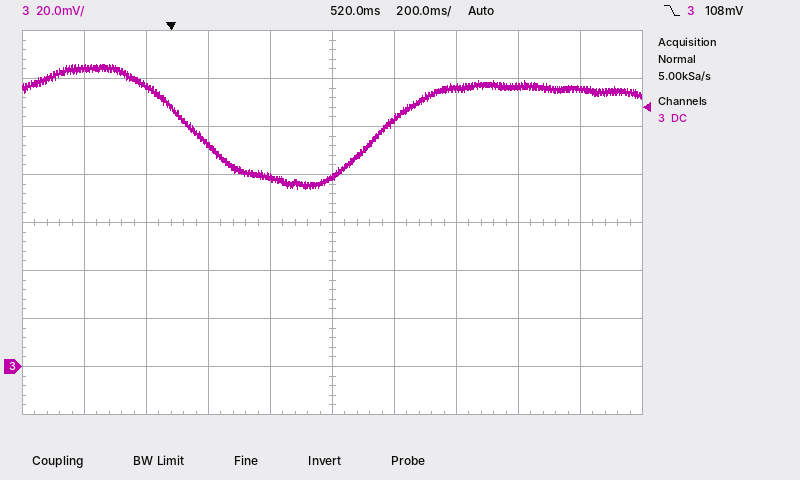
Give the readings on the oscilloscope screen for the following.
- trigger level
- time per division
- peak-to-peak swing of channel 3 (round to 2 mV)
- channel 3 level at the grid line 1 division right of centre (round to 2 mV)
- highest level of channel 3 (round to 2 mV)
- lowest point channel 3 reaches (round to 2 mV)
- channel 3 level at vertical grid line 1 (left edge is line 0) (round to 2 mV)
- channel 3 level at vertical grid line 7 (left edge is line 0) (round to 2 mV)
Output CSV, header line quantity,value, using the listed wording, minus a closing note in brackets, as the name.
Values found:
quantity,value
trigger level,108 mV
time per division,200 ms
peak-to-peak swing of channel 3,52 mV
channel 3 level at the grid line 1 division right of centre,104 mV
highest level of channel 3,126 mV
lowest point channel 3 reaches,74 mV
channel 3 level at vertical grid line 1 (left edge is line 0),124 mV
channel 3 level at vertical grid line 7 (left edge is line 0),116 mV
